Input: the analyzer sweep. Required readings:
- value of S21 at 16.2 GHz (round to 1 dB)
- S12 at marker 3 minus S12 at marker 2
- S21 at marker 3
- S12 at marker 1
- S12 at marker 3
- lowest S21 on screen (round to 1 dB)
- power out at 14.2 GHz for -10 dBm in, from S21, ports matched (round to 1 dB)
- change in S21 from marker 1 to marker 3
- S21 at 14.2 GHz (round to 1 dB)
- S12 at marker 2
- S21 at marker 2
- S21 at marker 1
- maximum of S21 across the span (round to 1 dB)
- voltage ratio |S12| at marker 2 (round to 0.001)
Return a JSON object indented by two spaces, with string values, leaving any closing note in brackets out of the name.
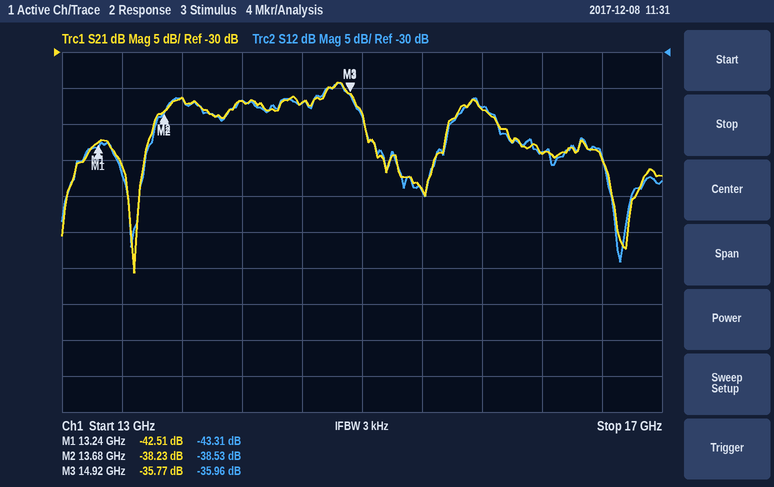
{
  "value of S21 at 16.2 GHz": "-44 dB",
  "S12 at marker 3 minus S12 at marker 2": "2.57 dB",
  "S21 at marker 3": "-35.77 dB",
  "S12 at marker 1": "-43.31 dB",
  "S12 at marker 3": "-35.96 dB",
  "lowest S21 on screen": "-61 dB",
  "power out at 14.2 GHz for -10 dBm in, from S21, ports matched": "-47 dBm",
  "change in S21 from marker 1 to marker 3": "6.74 dB",
  "S21 at 14.2 GHz": "-37 dB",
  "S12 at marker 2": "-38.53 dB",
  "S21 at marker 2": "-38.23 dB",
  "S21 at marker 1": "-42.51 dB",
  "maximum of S21 across the span": "-34 dB",
  "voltage ratio |S12| at marker 2": "0.012"
}
